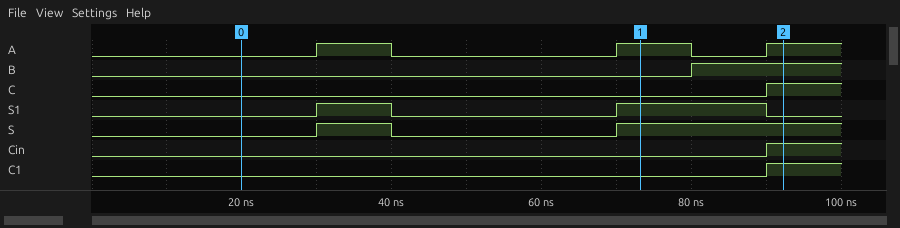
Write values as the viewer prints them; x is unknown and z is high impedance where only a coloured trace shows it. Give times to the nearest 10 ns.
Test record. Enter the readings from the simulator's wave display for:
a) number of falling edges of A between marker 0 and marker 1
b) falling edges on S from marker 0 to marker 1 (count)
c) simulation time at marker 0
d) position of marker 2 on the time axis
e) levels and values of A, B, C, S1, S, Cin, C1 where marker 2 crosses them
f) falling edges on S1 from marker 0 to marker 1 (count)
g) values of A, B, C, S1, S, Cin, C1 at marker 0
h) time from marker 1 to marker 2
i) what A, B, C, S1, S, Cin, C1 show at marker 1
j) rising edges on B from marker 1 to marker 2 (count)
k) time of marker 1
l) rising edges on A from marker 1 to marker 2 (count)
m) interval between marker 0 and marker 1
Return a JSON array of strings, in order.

["1", "1", "20 ns", "90 ns", "A=1, B=1, C=1, S1=0, S=1, Cin=1, C1=1", "1", "A=0, B=0, C=0, S1=0, S=0, Cin=0, C1=0", "20 ns", "A=1, B=0, C=0, S1=1, S=1, Cin=0, C1=0", "1", "70 ns", "1", "50 ns"]
